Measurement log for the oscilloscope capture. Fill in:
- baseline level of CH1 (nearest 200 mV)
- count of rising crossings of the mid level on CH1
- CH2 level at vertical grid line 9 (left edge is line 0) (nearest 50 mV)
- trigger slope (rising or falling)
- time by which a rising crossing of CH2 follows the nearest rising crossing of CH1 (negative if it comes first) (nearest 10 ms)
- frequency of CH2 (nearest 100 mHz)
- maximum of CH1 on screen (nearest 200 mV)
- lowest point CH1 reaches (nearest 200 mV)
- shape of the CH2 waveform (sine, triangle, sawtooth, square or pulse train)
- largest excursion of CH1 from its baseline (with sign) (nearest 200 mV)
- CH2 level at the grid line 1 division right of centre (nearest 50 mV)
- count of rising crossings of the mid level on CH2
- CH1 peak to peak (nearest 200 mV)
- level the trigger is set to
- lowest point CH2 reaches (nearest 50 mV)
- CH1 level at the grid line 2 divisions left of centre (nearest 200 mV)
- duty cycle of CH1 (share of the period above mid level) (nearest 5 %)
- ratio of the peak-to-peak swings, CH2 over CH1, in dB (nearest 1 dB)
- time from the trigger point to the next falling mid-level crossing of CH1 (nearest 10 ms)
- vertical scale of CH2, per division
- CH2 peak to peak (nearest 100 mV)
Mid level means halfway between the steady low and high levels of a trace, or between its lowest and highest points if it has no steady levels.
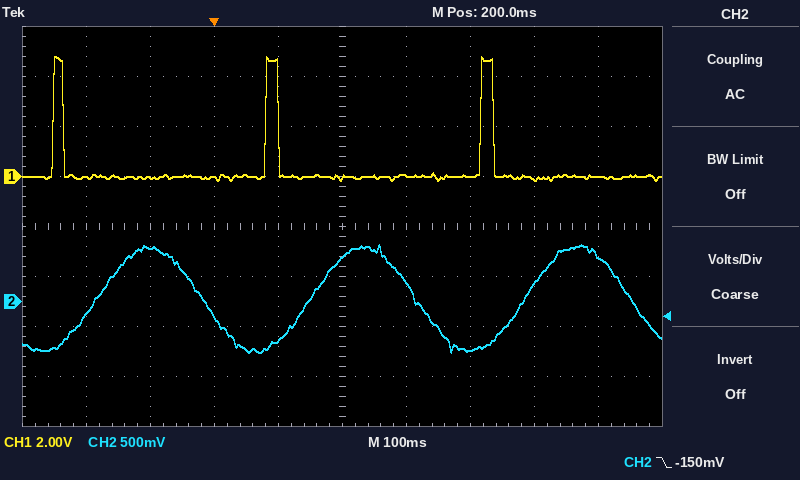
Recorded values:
0.0 V
3
450 mV
falling
+70 ms
3.0 Hz
4.8 V
-200 mV
sine
+4.8 V
200 mV
3
5.0 V
-150 mV
-500 mV
0.0 V
5 %
-13 dB
100 ms
500 mV
1.10 V
